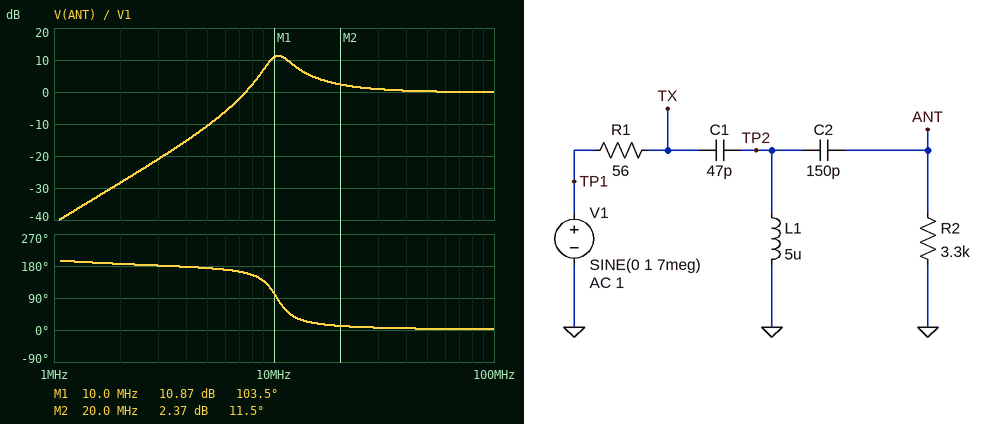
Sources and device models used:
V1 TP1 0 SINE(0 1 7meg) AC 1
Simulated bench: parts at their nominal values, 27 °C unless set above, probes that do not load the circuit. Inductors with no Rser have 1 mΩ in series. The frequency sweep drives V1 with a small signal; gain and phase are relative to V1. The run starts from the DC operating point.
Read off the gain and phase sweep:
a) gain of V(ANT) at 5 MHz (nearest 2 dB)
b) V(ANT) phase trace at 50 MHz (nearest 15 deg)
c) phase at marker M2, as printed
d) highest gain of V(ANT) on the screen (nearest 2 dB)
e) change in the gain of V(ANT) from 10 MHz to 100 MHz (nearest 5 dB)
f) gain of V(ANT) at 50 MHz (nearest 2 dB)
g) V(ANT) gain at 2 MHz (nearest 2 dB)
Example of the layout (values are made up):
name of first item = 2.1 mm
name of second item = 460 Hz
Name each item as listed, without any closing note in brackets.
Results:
gain of V(ANT) at 5 MHz = -10 dB
V(ANT) phase trace at 50 MHz = 0 deg
phase at marker M2, as printed = 11.5 deg
highest gain of V(ANT) on the screen = 12 dB
change in the gain of V(ANT) from 10 MHz to 100 MHz = -10 dB
gain of V(ANT) at 50 MHz = 0 dB
V(ANT) gain at 2 MHz = -28 dB
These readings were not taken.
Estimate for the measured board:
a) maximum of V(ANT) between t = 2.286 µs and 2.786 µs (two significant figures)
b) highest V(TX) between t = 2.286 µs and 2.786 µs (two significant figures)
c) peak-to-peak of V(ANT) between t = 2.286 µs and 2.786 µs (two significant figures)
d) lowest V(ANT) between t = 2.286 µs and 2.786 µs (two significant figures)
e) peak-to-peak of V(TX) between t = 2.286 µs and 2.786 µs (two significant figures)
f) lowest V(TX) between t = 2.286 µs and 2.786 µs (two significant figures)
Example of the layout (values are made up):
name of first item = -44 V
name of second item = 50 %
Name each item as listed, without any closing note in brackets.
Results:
maximum of V(ANT) between t = 2.286 µs and 2.786 µs = 800 mV
highest V(TX) between t = 2.286 µs and 2.786 µs = 970 mV
peak-to-peak of V(ANT) between t = 2.286 µs and 2.786 µs = 1.6 V
lowest V(ANT) between t = 2.286 µs and 2.786 µs = -800 mV
peak-to-peak of V(TX) between t = 2.286 µs and 2.786 µs = 1.9 V
lowest V(TX) between t = 2.286 µs and 2.786 µs = -970 mV
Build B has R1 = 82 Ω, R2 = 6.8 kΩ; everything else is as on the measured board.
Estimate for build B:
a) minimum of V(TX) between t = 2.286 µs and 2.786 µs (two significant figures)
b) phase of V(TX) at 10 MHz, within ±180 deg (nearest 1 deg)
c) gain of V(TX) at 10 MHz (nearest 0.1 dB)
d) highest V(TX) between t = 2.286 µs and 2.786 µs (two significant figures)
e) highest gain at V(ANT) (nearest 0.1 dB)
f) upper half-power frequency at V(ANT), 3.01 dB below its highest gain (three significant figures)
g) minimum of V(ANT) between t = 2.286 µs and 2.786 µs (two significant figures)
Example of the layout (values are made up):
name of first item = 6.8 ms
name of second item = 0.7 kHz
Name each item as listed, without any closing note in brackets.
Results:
minimum of V(TX) between t = 2.286 µs and 2.786 µs = -950 mV
phase of V(TX) at 10 MHz, within ±180 deg = -45 deg
gain of V(TX) at 10 MHz = -10.8 dB
highest V(TX) between t = 2.286 µs and 2.786 µs = 950 mV
highest gain at V(ANT) = 10.5 dB
upper half-power frequency at V(ANT), 3.01 dB below its highest gain = 12.7 MHz
minimum of V(ANT) between t = 2.286 µs and 2.786 µs = -790 mV
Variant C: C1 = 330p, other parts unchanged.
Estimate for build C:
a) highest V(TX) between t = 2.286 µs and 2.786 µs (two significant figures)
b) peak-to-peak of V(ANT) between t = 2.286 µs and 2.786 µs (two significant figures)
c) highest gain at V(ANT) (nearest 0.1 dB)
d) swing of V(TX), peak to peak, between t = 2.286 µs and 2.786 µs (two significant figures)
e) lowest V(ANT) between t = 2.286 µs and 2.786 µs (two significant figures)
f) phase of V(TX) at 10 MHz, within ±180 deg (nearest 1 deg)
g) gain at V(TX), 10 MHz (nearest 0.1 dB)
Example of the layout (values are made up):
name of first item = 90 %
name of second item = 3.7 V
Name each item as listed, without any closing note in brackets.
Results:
highest V(TX) between t = 2.286 µs and 2.786 µs = 910 mV
peak-to-peak of V(ANT) between t = 2.286 µs and 2.786 µs = 2.6 V
highest gain at V(ANT) = 6.3 dB
swing of V(TX), peak to peak, between t = 2.286 µs and 2.786 µs = 1.8 V
lowest V(ANT) between t = 2.286 µs and 2.786 µs = -1.3 V
phase of V(TX) at 10 MHz, within ±180 deg = 12 deg
gain at V(TX), 10 MHz = -0.4 dB
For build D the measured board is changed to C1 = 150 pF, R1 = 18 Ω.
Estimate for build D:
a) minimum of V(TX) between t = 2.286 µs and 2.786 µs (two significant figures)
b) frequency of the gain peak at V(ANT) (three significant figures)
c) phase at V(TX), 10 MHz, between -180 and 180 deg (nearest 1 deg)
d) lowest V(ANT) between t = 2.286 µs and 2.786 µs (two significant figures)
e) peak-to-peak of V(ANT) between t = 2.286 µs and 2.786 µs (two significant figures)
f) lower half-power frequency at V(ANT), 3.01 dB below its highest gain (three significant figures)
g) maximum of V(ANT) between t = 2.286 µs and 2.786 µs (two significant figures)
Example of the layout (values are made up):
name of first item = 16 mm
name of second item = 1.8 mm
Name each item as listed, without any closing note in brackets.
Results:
minimum of V(TX) between t = 2.286 µs and 2.786 µs = -920 mV
frequency of the gain peak at V(ANT) = 5.82 MHz
phase at V(TX), 10 MHz, between -180 and 180 deg = 5 deg
lowest V(ANT) between t = 2.286 µs and 2.786 µs = -2.9 V
peak-to-peak of V(ANT) between t = 2.286 µs and 2.786 µs = 5.8 V
lower half-power frequency at V(ANT), 3.01 dB below its highest gain = 5.42 MHz
maximum of V(ANT) between t = 2.286 µs and 2.786 µs = 2.9 V
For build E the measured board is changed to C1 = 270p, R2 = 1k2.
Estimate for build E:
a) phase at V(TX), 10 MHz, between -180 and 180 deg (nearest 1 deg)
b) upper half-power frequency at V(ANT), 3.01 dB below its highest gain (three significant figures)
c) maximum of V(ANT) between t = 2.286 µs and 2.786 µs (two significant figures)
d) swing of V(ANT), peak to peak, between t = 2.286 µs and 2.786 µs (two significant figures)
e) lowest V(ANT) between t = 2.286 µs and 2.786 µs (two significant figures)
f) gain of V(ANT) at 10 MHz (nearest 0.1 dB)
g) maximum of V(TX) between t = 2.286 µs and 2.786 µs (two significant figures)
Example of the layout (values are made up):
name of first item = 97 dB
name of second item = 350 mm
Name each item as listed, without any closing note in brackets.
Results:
phase at V(TX), 10 MHz, between -180 and 180 deg = 11 deg
upper half-power frequency at V(ANT), 3.01 dB below its highest gain = 6.85 MHz
maximum of V(ANT) between t = 2.286 µs and 2.786 µs = 1.3 V
swing of V(ANT), peak to peak, between t = 2.286 µs and 2.786 µs = 2.7 V
lowest V(ANT) between t = 2.286 µs and 2.786 µs = -1.3 V
gain of V(ANT) at 10 MHz = 1.0 dB
maximum of V(TX) between t = 2.286 µs and 2.786 µs = 850 mV
